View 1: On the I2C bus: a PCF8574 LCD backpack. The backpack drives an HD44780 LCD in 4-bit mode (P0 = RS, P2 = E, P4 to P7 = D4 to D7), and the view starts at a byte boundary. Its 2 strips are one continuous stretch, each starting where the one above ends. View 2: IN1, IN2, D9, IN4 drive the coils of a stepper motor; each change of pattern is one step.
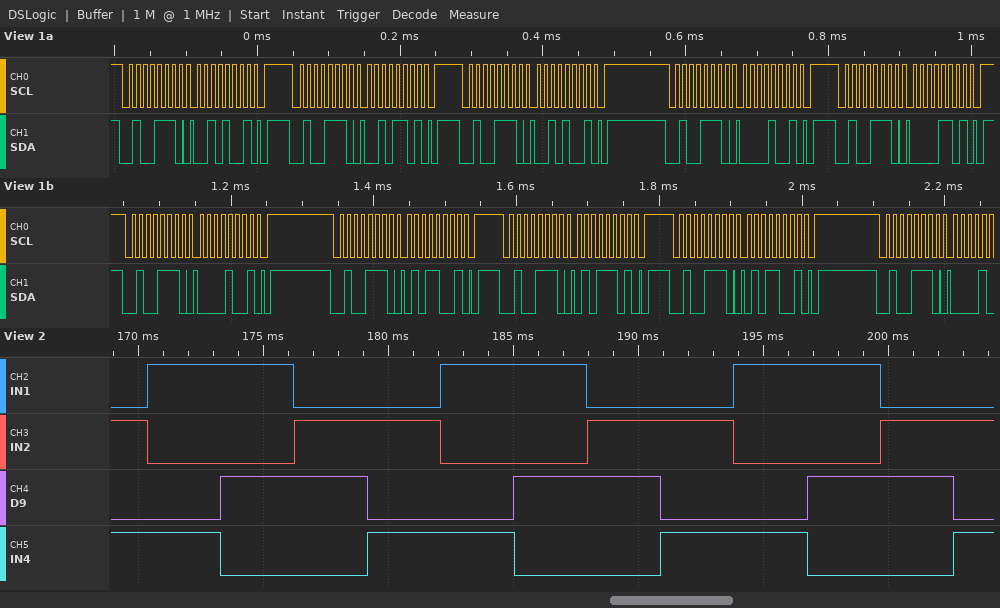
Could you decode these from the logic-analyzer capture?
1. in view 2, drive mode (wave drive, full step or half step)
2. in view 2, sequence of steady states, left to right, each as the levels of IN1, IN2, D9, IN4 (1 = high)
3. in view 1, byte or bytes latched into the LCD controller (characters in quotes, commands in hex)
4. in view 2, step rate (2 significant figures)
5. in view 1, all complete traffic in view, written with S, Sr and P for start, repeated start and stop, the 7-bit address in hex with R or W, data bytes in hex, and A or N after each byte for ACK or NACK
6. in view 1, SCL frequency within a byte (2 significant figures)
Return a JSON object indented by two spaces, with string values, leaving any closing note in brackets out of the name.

{
  "in view 2, drive mode": "full step",
  "in view 2, sequence of steady states, left to right, each as the levels of IN1, IN2, D9, IN4": "0101 1001 1010 0110 0101 1001 1010 0110 0101 1001 1010 0110 0101",
  "in view 1, byte or bytes latched into the LCD controller": "' '",
  "in view 2, step rate": "340 steps/s",
  "in view 1, all complete traffic in view, written with S, Sr and P for start, repeated start and stop, the 7-bit address in hex with R or W, data bytes in hex, and A or N after each byte for ACK or NACK": "S 27W A 29 A P S 27W A 2D A P S 27W A 29 A P S 27W A 09 A P S 27W A 0D A P S 27W A 09 A P S 27W A 59 A P S 27W A 5D A P S 27W A 59 A P S 27W A",
  "in view 1, SCL frequency within a byte": "100 kHz"
}
